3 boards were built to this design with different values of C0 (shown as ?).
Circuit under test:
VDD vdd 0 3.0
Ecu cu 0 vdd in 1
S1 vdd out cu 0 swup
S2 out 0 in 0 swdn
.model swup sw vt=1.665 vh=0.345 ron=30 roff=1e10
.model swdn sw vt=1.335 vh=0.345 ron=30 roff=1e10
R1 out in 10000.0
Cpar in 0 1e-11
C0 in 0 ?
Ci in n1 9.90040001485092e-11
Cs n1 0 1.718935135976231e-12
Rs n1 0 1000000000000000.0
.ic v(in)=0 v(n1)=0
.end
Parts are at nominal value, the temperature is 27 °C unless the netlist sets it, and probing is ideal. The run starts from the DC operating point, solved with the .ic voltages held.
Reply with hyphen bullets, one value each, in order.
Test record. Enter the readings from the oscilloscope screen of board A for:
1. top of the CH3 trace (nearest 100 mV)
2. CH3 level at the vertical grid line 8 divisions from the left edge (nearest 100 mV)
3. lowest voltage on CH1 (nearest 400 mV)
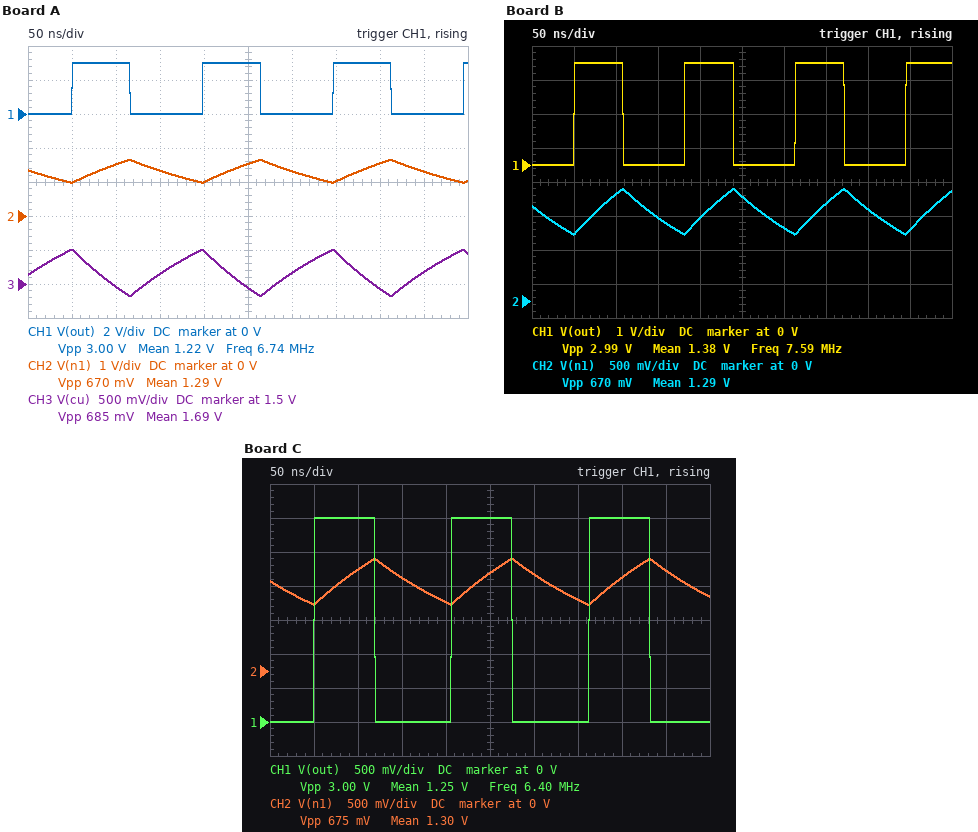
- 2.0 V
- 1.4 V
- 0 V
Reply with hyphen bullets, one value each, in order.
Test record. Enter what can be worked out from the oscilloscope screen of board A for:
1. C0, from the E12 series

- 3.9 pF
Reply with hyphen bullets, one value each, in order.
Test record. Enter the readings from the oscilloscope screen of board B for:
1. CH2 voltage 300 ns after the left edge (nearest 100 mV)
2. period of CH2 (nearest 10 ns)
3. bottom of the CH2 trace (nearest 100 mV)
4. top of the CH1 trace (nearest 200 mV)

- 1.1 V
- 130 ns
- 1.0 V
- 3.0 V
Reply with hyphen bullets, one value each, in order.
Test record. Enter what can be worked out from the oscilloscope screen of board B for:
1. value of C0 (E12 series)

- 2.2 pF
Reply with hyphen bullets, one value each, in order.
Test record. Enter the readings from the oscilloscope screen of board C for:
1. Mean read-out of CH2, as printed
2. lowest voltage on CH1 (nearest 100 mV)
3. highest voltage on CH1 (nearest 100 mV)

- 1.30 V
- 0 V
- 3.0 V
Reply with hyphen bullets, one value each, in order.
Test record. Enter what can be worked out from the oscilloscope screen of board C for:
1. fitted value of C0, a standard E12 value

- 4.7 pF
